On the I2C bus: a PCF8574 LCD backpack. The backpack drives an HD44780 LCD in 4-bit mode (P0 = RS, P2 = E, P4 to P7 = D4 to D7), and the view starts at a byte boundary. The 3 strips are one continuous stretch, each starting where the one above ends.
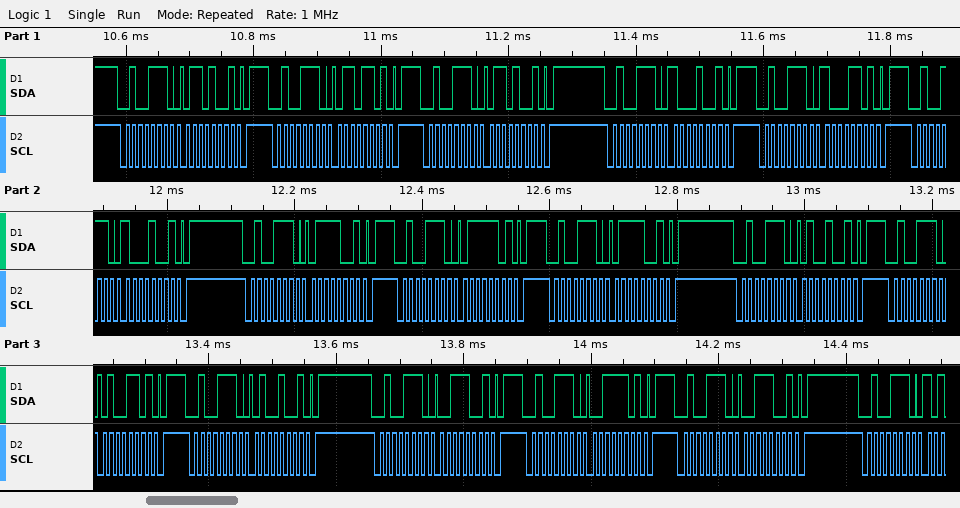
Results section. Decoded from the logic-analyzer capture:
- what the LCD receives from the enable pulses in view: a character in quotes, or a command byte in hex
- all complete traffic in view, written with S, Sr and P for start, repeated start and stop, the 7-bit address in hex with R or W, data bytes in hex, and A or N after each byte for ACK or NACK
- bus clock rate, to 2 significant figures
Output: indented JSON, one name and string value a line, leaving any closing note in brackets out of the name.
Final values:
{
  "what the LCD receives from the enable pulses in view: a character in quotes, or a command byte in hex": "'h' 't'",
  "all complete traffic in view, written with S, Sr and P for start, repeated start and stop, the 7-bit address in hex with R or W, data bytes in hex, and A or N after each byte for ACK or NACK": "S 27W A 69 A P S 27W A 6D A P S 27W A 69 A P S 27W A 89 A P S 27W A 8D A P S 27W A 89 A P S 27W A 79 A P S 27W A 7D A P S 27W A 79 A P S 27W A 49 A P S 27W A 4D A P S 27W A 49 A P S 27W A 39 A P S 27W A 3D A P S 27W A 39 A P S 27W A",
  "bus clock rate, to 2 significant figures": "100 kHz"
}
